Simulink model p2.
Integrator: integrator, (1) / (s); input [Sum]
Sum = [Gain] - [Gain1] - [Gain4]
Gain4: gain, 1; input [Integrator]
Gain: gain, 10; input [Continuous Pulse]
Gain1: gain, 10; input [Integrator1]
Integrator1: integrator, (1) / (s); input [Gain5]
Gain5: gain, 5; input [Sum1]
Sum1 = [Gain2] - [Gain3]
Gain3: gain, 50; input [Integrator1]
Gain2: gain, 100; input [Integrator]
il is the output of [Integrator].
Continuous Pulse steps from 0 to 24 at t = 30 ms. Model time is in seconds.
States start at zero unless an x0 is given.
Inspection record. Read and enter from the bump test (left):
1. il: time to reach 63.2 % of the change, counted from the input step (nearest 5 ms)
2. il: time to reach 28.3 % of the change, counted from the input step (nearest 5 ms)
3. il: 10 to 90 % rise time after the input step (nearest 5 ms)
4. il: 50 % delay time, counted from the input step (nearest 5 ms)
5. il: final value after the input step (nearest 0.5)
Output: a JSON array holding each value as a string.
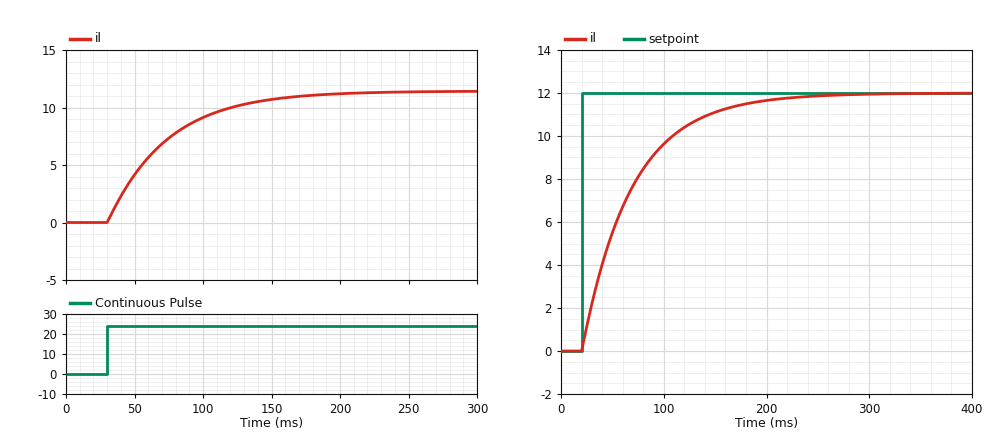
["45 ms", "15 ms", "95 ms", "30 ms", "11.5"]
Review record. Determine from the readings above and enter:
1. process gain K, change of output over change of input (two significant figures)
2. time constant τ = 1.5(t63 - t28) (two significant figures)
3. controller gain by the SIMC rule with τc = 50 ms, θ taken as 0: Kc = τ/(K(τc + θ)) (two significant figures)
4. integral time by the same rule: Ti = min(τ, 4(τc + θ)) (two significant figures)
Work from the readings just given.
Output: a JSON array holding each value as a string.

["0.48", "45 ms", "1.9", "45 ms"]
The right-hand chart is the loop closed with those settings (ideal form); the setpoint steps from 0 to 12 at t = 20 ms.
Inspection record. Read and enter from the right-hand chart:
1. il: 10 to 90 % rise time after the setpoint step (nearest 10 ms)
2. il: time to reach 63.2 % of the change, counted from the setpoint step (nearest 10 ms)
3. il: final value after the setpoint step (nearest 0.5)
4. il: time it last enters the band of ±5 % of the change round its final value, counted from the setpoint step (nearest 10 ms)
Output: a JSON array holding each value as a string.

["110 ms", "50 ms", "12.0", "150 ms"]
